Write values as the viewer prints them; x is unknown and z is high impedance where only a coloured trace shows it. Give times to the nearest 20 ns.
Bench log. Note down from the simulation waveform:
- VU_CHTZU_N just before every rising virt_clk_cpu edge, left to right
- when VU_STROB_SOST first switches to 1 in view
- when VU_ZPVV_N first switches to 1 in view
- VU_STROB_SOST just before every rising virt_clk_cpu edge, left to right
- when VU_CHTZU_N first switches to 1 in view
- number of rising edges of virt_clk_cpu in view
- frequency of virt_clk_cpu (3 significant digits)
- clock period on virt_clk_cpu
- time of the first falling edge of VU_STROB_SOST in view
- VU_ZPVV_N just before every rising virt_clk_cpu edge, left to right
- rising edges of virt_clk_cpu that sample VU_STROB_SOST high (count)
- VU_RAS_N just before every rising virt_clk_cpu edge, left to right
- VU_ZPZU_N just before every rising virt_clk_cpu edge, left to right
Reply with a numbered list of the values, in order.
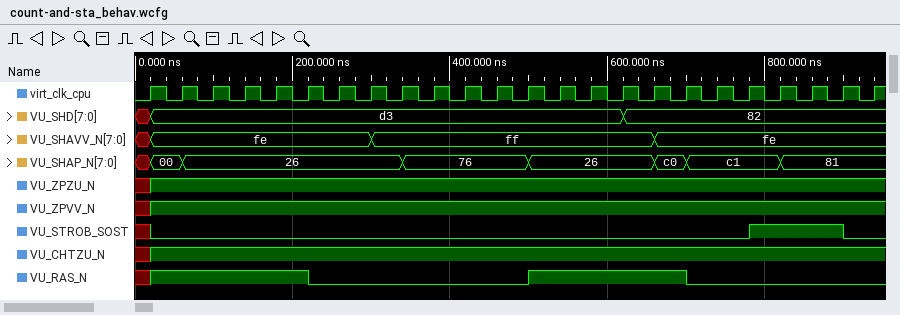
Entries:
1. x 1 1 1 1 1 1 1 1 1 1 1 1 1 1 1 1 1 1 1 1 1 1 1
2. 780 ns
3. 20 ns
4. x 0 0 0 0 0 0 0 0 0 0 0 0 0 0 0 0 0 0 0 1 1 1 0
5. 20 ns
6. 24
7. 25.0 MHz
8. 40 ns
9. 900 ns
10. x 1 1 1 1 1 1 1 1 1 1 1 1 1 1 1 1 1 1 1 1 1 1 1
11. 3
12. x 1 1 1 1 1 0 0 0 0 0 0 0 1 1 1 1 1 0 0 0 0 0 0
13. x 1 1 1 1 1 1 1 1 1 1 1 1 1 1 1 1 1 1 1 1 1 1 1
